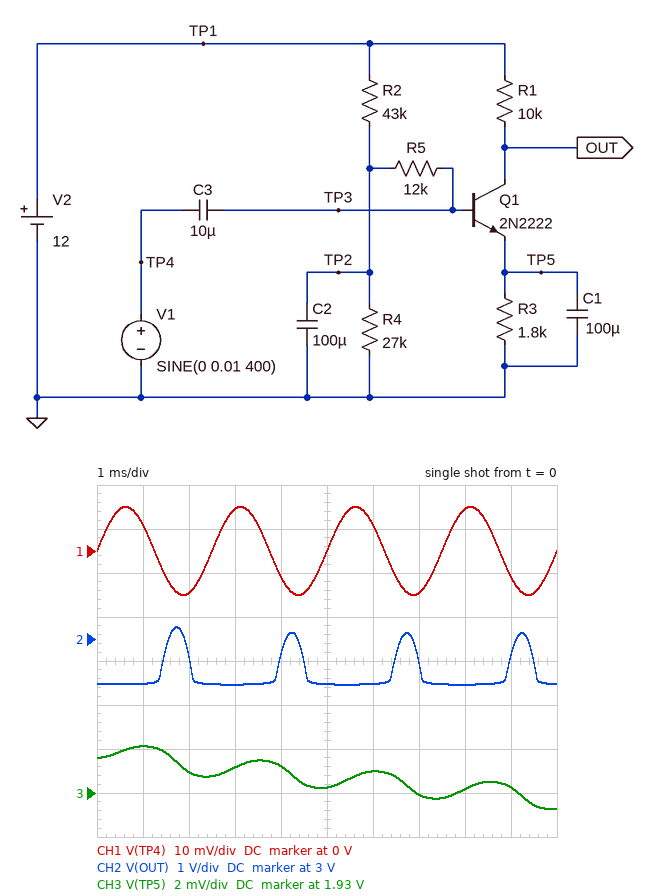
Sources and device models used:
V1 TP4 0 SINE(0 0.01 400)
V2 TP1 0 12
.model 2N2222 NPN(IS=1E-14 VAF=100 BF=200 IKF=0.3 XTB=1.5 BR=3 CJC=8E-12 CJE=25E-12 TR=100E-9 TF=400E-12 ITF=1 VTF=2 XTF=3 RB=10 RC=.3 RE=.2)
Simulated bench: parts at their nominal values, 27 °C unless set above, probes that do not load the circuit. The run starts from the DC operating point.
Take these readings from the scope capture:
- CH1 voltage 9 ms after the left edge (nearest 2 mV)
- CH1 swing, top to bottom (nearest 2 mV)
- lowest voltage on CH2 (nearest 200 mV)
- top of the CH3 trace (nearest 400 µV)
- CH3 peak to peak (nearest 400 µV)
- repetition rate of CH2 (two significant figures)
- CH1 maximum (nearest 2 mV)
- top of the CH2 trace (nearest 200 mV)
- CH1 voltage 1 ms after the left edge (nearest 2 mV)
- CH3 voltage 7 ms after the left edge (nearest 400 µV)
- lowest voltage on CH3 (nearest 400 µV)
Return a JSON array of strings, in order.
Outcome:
["-6 mV", "20 mV", "2.0 V", "1.9320 V", "2.8 mV", "400 Hz", "10 mV", "3.2 V", "6 mV", "1.9300 V", "1.9292 V"]
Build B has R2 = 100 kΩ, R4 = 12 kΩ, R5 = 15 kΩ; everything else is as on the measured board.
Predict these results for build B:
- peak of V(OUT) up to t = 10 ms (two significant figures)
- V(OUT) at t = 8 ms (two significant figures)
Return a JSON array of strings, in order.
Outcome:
["9.7 V", "7.2 V"]
